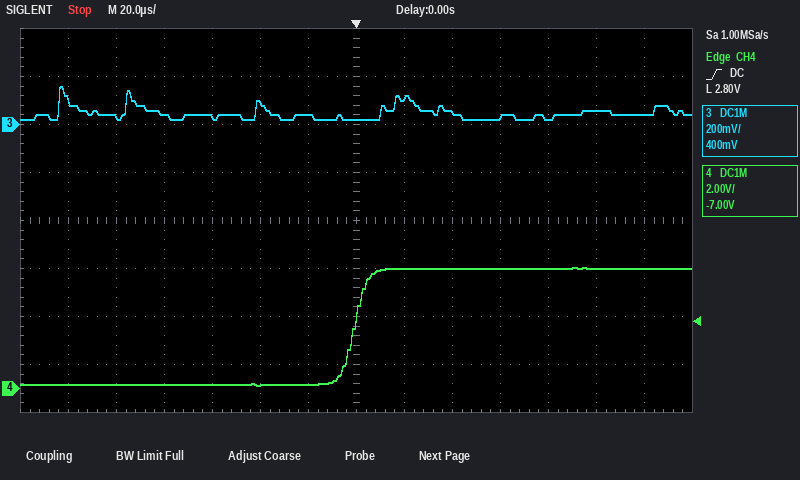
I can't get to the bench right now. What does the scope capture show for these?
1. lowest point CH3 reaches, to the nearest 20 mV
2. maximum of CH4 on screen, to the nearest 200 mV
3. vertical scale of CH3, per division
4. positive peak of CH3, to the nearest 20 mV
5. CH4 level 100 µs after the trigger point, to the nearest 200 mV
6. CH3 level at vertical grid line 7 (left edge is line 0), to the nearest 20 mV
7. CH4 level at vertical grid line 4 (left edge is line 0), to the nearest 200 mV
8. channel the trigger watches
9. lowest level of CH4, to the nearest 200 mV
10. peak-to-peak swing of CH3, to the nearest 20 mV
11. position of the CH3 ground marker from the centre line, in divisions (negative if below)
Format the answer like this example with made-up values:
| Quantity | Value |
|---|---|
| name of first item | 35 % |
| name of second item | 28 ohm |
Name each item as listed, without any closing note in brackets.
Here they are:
| Quantity | Value |
|---|---|
| lowest point CH3 reaches, to the nearest 20 mV | 20 mV |
| maximum of CH4 on screen, to the nearest 200 mV | 5.0 V |
| vertical scale of CH3, per division | 200 mV |
| positive peak of CH3, to the nearest 20 mV | 160 mV |
| CH4 level 100 µs after the trigger point, to the nearest 200 mV | 5.0 V |
| CH3 level at vertical grid line 7 (left edge is line 0), to the nearest 20 mV | 20 mV |
| CH4 level at vertical grid line 4 (left edge is line 0), to the nearest 200 mV | 200 mV |
| channel the trigger watches | CH4 |
| lowest level of CH4, to the nearest 200 mV | 200 mV |
| peak-to-peak swing of CH3, to the nearest 20 mV | 140 mV |
| position of the CH3 ground marker from the centre line, in divisions | +2.0 div |
